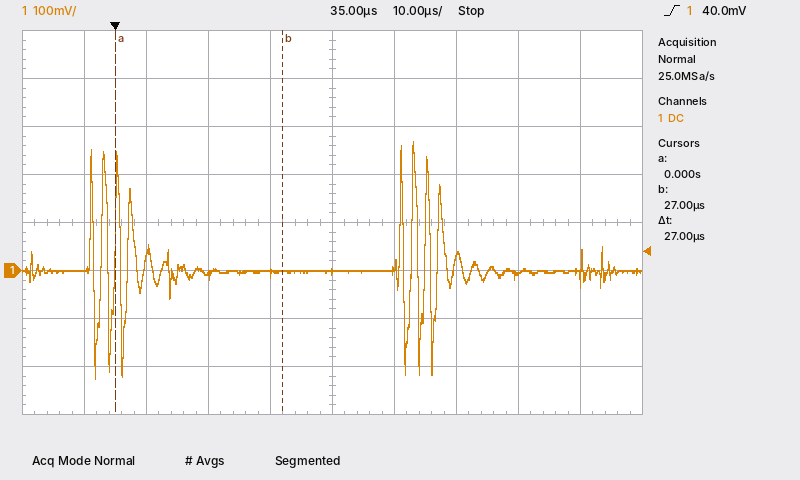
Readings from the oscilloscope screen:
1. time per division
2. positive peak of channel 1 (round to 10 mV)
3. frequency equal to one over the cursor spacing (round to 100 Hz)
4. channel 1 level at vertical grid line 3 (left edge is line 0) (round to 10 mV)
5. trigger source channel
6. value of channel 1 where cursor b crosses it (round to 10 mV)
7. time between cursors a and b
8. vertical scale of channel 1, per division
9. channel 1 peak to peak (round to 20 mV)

10 µs
270 mV
37.0 kHz
-10 mV
channel 1
0 mV
27 µs
100 mV
500 mV
